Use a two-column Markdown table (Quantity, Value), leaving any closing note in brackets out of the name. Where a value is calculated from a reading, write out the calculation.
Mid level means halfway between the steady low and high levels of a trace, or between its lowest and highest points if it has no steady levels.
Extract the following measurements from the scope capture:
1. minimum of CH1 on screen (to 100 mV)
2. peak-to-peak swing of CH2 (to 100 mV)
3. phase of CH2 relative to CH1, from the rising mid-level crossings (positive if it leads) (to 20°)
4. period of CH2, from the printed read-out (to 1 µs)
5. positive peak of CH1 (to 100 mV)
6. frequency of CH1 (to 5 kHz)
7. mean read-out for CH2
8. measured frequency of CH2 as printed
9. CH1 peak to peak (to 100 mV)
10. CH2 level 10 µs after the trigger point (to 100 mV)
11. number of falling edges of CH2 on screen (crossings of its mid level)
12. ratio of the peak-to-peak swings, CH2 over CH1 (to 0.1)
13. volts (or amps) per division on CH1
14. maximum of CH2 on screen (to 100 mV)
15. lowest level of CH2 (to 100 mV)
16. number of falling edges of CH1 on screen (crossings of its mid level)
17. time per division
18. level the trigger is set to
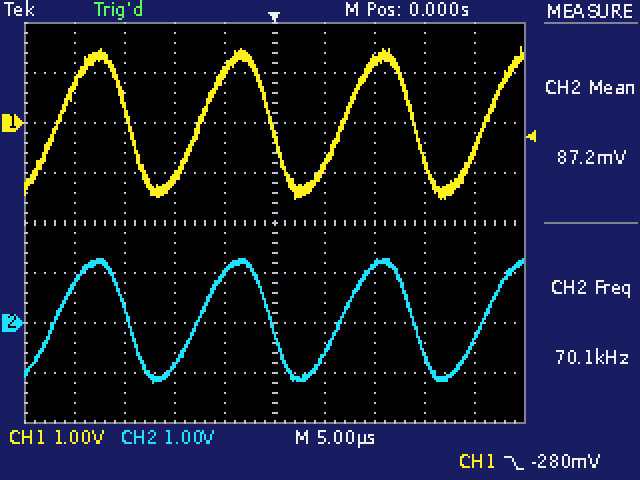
| Quantity | Value |
|---|---|
| minimum of CH1 on screen | -1.5 V |
| peak-to-peak swing of CH2 | 1.3 V − (-1.2 V) = 2.5 V |
| phase of CH2 relative to CH1, from the rising mid-level crossings (positive if it leads) | 0° |
| period of CH2, from the printed read-out | 1 / 70.1 kHz ≈ 14 µs |
| positive peak of CH1 | 1.5 V |
| frequency of CH1 | 70 kHz |
| mean read-out for CH2 | 87.2 mV |
| measured frequency of CH2 as printed | 70.1 kHz |
| CH1 peak to peak | 1.5 V − (-1.5 V) = 3.0 V |
| CH2 level 10 µs after the trigger point | 1.2 V |
| number of falling edges of CH2 on screen | 3 |
| ratio of the peak-to-peak swings, CH2 over CH1 | 2.5 V / 3.0 V ≈ 0.8 |
| volts (or amps) per division on CH1 | 1 V |
| maximum of CH2 on screen | 1.3 V |
| lowest level of CH2 | -1.2 V |
| number of falling edges of CH1 on screen | 3 |
| time per division | 5 µs |
| level the trigger is set to | -280 mV |
